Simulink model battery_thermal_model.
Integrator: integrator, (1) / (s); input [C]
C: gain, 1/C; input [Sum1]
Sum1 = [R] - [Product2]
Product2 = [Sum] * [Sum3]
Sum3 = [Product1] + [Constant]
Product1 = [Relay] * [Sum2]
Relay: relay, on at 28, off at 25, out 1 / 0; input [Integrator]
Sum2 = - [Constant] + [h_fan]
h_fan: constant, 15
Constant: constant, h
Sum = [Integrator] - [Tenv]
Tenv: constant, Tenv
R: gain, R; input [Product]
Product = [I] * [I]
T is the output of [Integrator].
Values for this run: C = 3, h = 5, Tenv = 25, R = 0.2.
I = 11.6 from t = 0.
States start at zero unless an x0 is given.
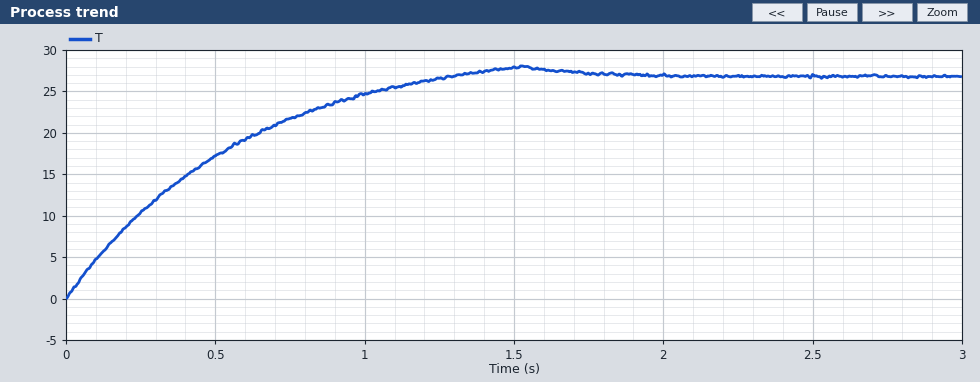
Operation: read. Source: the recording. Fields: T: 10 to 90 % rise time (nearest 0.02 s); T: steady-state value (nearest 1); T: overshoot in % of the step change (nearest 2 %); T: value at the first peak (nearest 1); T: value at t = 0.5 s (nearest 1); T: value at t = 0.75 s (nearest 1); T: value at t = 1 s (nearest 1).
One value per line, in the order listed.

0.90 s
27
4 %
28
17
22
25
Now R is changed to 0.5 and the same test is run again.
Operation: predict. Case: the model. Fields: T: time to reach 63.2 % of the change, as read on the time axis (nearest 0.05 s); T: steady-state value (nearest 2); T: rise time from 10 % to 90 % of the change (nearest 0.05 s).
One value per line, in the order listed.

0.40 s
30
0.65 s
